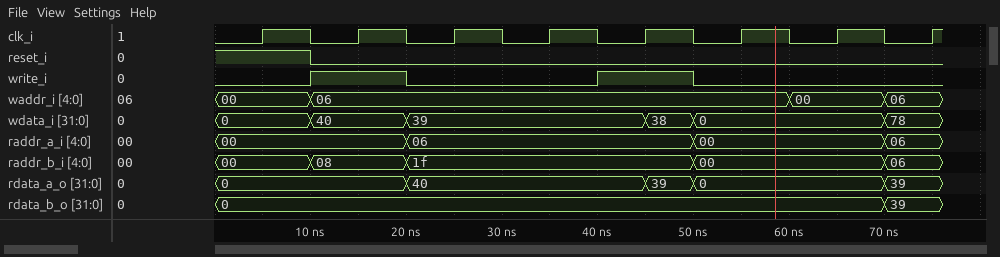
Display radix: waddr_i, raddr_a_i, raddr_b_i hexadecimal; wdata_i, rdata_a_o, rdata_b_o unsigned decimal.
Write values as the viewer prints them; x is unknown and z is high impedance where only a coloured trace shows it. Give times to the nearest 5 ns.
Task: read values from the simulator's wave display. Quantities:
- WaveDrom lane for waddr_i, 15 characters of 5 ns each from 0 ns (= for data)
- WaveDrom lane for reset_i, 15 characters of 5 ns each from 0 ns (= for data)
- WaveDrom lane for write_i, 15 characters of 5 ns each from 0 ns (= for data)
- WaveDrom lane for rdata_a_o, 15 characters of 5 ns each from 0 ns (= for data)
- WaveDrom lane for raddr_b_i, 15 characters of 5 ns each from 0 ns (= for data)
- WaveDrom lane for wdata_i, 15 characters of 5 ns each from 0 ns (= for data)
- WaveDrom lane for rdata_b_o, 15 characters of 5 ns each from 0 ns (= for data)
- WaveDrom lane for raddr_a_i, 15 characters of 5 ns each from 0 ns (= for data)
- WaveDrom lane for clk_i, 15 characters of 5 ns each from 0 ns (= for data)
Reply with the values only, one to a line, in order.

{name: 'waddr_i', wave: '=.=.........=.=', data: '00 06 00 06'}
{name: 'reset_i', wave: '1.0............'}
{name: 'write_i', wave: '0.1.0...1.0....'}
{name: 'rdata_a_o', wave: '=...=....==...=', data: '0 40 39 0 39'}
{name: 'raddr_b_i', wave: '=.=.=.....=...=', data: '00 08 1f 00 06'}
{name: 'wdata_i', wave: '=.=.=....==...=', data: '0 40 39 38 0 78'}
{name: 'rdata_b_o', wave: '=.............=', data: '0 39'}
{name: 'raddr_a_i', wave: '=...=.....=...=', data: '00 06 00 06'}
{name: 'clk_i', wave: '010101010101010'}
